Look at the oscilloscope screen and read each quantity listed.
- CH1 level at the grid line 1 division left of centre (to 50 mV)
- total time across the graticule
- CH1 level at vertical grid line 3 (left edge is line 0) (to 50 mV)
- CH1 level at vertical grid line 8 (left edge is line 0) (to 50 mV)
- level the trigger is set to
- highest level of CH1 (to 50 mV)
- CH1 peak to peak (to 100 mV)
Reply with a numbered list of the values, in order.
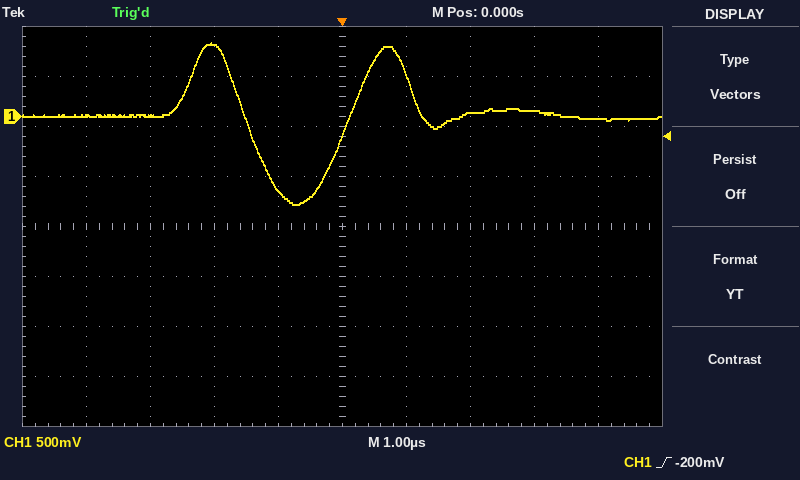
1. -750 mV
2. 10 µs
3. 700 mV
4. 50 mV
5. -200 mV
6. 750 mV
7. 1.60 V
